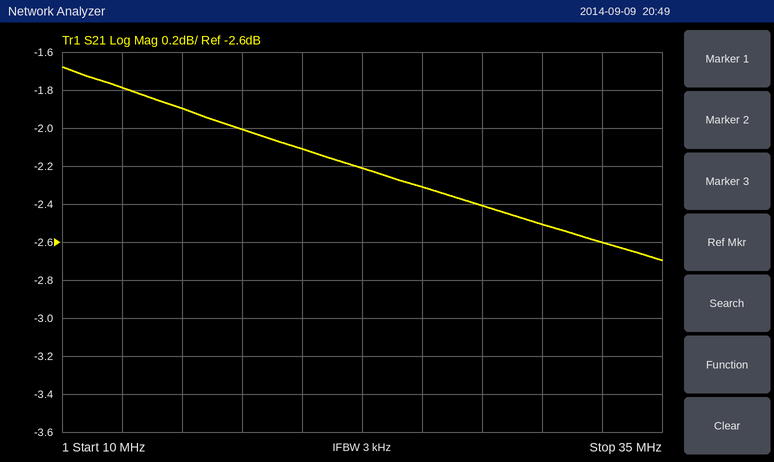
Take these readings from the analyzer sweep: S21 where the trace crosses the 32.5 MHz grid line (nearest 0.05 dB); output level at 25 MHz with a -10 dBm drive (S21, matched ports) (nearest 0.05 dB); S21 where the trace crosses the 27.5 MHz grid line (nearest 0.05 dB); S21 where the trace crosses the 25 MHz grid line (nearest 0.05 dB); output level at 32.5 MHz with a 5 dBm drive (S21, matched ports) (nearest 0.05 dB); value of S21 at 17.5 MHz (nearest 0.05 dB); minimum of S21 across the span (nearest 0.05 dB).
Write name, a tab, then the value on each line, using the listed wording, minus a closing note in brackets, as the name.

S21 where the trace crosses the 32.5 MHz grid line	-2.60 dB
output level at 25 MHz with a -10 dBm drive (S21, matched ports)	-12.30 dBm
S21 where the trace crosses the 27.5 MHz grid line	-2.40 dB
S21 where the trace crosses the 25 MHz grid line	-2.30 dB
output level at 32.5 MHz with a 5 dBm drive (S21, matched ports)	2.40 dBm
value of S21 at 17.5 MHz	-2.00 dB
minimum of S21 across the span	-2.70 dB
